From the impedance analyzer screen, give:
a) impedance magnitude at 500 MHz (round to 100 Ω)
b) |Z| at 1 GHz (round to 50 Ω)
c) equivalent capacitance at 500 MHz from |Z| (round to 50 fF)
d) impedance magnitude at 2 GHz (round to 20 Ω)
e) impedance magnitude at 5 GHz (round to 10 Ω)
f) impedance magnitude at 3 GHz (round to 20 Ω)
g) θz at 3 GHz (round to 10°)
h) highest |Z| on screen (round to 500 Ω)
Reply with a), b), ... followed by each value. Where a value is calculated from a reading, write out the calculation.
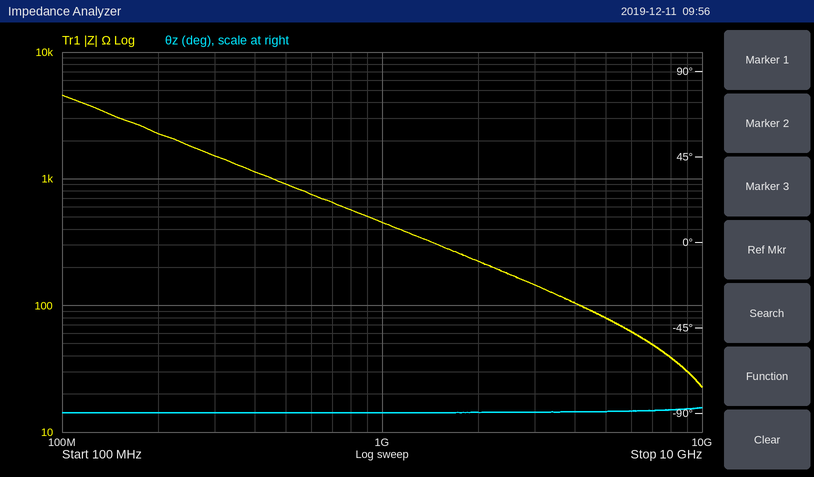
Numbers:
a) 900 Ω
b) 450 Ω
c) C = 1/(2π × 500 MHz × 900 Ω) ≈ 354 fF, so 350 fF to the nearest 50 fF
d) 220 Ω
e) 80 Ω
f) 140 Ω
g) -90°
h) 4.5 kΩ
